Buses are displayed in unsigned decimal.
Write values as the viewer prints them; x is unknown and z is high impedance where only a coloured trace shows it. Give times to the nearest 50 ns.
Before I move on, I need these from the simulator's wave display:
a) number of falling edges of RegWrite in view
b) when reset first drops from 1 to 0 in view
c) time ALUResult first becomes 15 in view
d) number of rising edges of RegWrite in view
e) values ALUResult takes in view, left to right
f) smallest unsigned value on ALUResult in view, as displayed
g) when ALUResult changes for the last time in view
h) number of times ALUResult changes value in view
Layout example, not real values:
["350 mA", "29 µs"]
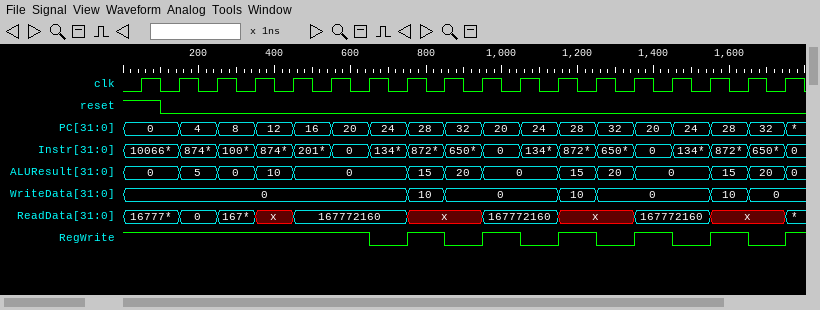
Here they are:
["6", "100 ns", "750 ns", "6", "0, 5, 0, 10, 0, 15, 20, 0, 15, 20, 0, 15, 20, 0", "0", "1750 ns", "13"]
